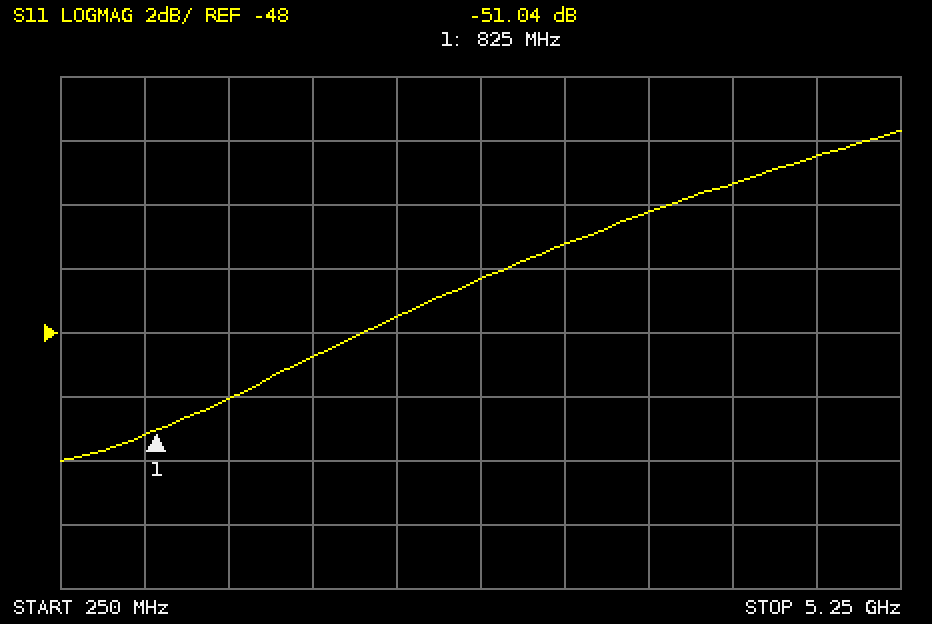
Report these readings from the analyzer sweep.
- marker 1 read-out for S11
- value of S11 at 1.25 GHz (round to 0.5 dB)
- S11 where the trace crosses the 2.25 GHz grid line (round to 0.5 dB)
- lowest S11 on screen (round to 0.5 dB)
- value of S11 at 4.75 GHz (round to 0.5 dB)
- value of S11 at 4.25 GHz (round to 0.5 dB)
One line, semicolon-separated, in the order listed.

-51.04 dB; -50.0 dB; -47.5 dB; -52.0 dB; -42.5 dB; -43.5 dB
